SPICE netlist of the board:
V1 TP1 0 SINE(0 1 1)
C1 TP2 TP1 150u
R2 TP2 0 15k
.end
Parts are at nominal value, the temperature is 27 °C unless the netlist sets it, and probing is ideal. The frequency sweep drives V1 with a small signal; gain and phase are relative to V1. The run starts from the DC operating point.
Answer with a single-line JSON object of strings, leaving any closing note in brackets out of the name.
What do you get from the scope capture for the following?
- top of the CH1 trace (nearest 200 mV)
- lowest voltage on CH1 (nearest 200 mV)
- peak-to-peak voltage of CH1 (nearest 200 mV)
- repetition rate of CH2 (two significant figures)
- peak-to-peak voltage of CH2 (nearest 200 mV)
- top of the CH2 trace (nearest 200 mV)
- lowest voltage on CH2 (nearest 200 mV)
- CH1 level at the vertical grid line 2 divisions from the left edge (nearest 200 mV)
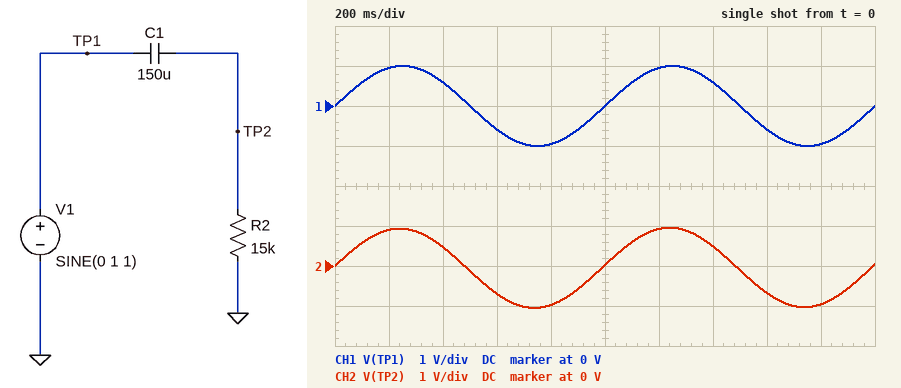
{"top of the CH1 trace": "1.0 V", "lowest voltage on CH1": "-1.0 V", "peak-to-peak voltage of CH1": "2.0 V", "repetition rate of CH2": "1.0 Hz", "peak-to-peak voltage of CH2": "2.0 V", "top of the CH2 trace": "1.0 V", "lowest voltage on CH2": "-1.0 V", "CH1 level at the vertical grid line 2 divisions from the left edge": "600 mV"}
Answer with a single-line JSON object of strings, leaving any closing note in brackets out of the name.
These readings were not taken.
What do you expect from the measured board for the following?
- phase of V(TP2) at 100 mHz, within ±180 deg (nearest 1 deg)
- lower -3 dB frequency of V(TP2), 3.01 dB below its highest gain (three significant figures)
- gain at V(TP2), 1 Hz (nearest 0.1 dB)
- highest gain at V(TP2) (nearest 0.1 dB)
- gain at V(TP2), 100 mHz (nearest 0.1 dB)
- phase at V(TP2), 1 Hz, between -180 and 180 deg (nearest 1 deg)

{"phase of V(TP2) at 100 mHz, within ±180 deg": "35 deg", "lower -3 dB frequency of V(TP2), 3.01 dB below its highest gain": "70.7 mHz", "gain at V(TP2), 1 Hz": "0 dB", "highest gain at V(TP2)": "0 dB", "gain at V(TP2), 100 mHz": "-1.8 dB", "phase at V(TP2), 1 Hz, between -180 and 180 deg": "4 deg"}
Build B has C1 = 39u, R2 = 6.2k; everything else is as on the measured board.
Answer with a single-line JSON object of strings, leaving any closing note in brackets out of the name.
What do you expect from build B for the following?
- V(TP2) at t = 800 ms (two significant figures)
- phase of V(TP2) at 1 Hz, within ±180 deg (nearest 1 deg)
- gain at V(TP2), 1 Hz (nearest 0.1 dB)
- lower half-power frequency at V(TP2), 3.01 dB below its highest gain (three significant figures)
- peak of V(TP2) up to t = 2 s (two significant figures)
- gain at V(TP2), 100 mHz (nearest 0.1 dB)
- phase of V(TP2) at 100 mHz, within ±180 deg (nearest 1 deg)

{"V(TP2) at t = 800 ms": "-540 mV", "phase of V(TP2) at 1 Hz, within ±180 deg": "33 deg", "gain at V(TP2), 1 Hz": "-1.6 dB", "lower half-power frequency at V(TP2), 3.01 dB below its highest gain": "658 mHz", "peak of V(TP2) up to t = 2 s": "830 mV", "gain at V(TP2), 100 mHz": "-16.5 dB", "phase of V(TP2) at 100 mHz, within ±180 deg": "81 deg"}
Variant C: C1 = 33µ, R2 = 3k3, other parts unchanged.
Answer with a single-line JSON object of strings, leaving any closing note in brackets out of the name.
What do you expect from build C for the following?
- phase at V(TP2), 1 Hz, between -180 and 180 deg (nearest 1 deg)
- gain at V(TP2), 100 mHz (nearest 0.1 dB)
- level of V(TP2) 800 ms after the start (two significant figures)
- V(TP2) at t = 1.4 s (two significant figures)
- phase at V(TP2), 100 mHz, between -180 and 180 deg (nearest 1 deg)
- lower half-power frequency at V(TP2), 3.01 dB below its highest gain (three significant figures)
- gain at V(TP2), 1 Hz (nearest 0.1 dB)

{"phase at V(TP2), 1 Hz, between -180 and 180 deg": "56 deg", "gain at V(TP2), 100 mHz": "-23.3 dB", "level of V(TP2) 800 ms after the start": "-160 mV", "V(TP2) at t = 1.4 s": "-190 mV", "phase at V(TP2), 100 mHz, between -180 and 180 deg": "86 deg", "lower half-power frequency at V(TP2), 3.01 dB below its highest gain": "1.46 Hz", "gain at V(TP2), 1 Hz": "-5.0 dB"}
